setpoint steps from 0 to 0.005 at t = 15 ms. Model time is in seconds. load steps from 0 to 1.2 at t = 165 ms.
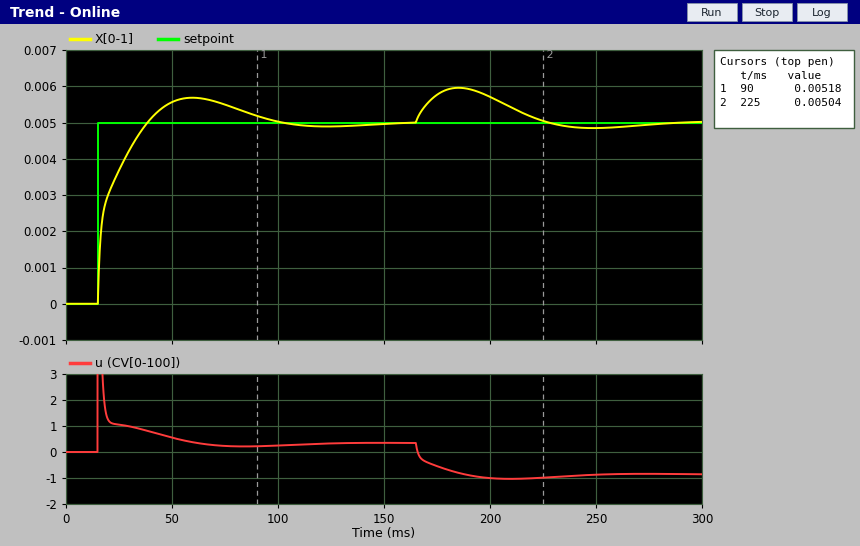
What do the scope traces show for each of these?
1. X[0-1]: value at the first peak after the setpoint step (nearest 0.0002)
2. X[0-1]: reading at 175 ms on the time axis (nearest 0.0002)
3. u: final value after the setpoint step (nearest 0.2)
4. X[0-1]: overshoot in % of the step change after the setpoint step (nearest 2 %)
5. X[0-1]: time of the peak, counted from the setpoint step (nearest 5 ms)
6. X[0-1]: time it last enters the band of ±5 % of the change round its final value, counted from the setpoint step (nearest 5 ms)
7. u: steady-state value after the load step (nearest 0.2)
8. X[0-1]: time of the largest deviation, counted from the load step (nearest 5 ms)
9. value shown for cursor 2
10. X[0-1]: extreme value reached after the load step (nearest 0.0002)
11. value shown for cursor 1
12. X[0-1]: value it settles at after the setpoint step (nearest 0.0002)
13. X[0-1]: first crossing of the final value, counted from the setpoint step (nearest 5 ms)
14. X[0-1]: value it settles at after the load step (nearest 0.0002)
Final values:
0.0056
0.0058
0.4
14 %
45 ms
70 ms
-0.8
20 ms
0.00504
0.0060
0.00518
0.0050
25 ms
0.0050
